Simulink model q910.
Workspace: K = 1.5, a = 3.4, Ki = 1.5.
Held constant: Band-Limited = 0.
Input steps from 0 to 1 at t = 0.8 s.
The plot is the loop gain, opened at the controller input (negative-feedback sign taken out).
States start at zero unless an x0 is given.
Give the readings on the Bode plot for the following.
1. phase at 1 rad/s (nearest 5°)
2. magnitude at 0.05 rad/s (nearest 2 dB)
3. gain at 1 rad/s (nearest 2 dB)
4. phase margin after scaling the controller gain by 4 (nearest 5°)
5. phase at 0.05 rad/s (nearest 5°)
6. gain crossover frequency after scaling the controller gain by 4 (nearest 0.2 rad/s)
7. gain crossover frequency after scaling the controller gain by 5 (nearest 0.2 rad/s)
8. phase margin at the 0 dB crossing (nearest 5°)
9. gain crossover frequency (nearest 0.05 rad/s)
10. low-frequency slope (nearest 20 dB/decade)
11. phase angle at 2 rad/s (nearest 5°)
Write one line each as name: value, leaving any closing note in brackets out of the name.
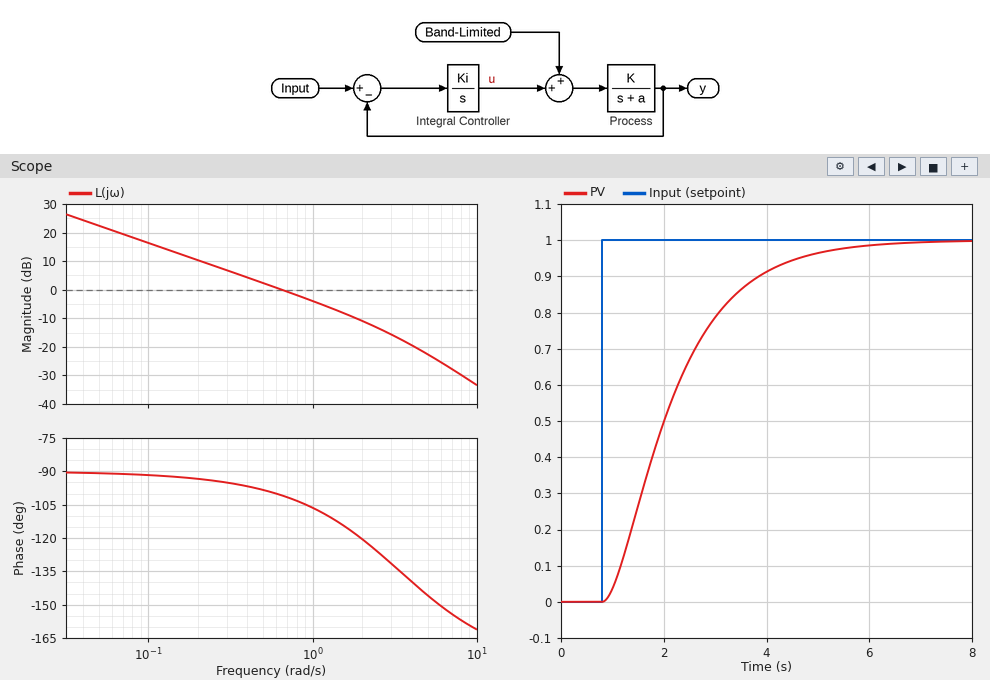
phase at 1 rad/s: -105°
magnitude at 0.05 rad/s: 22 dB
gain at 1 rad/s: -4 dB
phase margin after scaling the controller gain by 4: 55°
phase at 0.05 rad/s: -90°
gain crossover frequency after scaling the controller gain by 4: 2.2 rad/s
gain crossover frequency after scaling the controller gain by 5: 2.6 rad/s
phase margin at the 0 dB crossing: 80°
gain crossover frequency: 0.65 rad/s
low-frequency slope: -20 dB/decade
phase angle at 2 rad/s: -120°
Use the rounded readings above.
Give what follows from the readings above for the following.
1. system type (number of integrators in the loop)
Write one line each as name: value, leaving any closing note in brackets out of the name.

system type: 1
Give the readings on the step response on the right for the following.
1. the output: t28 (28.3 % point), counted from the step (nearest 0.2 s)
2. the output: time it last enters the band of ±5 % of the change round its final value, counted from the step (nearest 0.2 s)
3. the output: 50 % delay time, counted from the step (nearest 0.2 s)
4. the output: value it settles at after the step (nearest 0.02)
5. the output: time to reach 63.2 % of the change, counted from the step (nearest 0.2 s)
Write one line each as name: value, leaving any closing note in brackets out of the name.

the output: t28 (28.3 % point), counted from the step: 0.8 s
the output: time it last enters the band of ±5 % of the change round its final value, counted from the step: 3.8 s
the output: 50 % delay time, counted from the step: 1.2 s
the output: value it settles at after the step: 1.00
the output: time to reach 63.2 % of the change, counted from the step: 1.6 s
